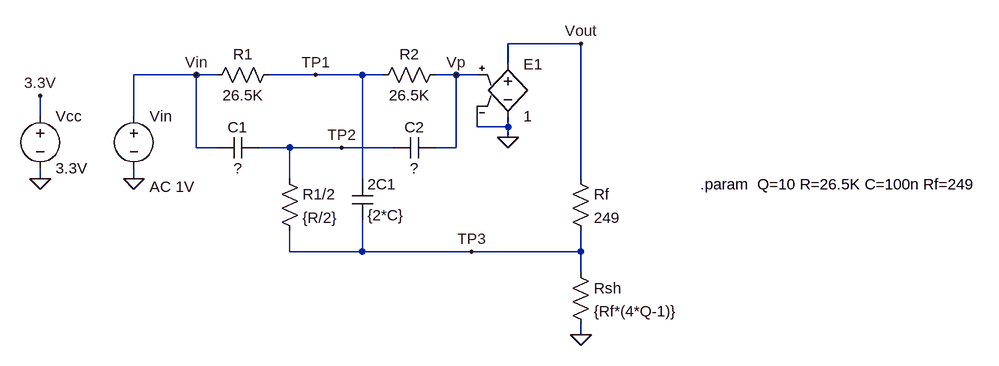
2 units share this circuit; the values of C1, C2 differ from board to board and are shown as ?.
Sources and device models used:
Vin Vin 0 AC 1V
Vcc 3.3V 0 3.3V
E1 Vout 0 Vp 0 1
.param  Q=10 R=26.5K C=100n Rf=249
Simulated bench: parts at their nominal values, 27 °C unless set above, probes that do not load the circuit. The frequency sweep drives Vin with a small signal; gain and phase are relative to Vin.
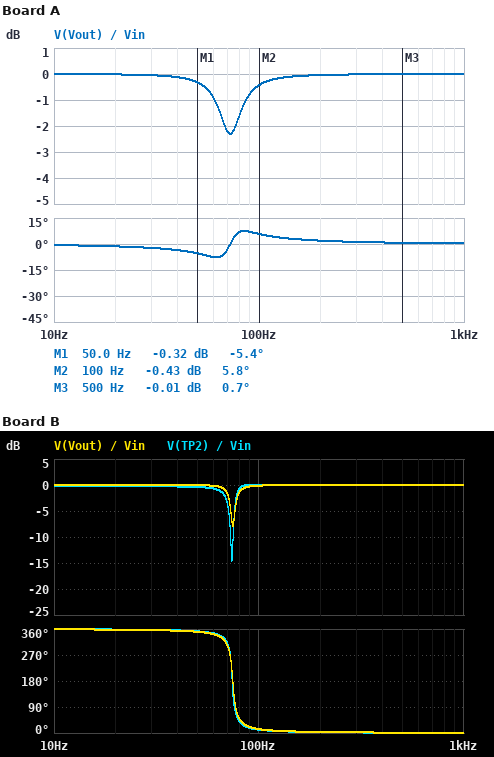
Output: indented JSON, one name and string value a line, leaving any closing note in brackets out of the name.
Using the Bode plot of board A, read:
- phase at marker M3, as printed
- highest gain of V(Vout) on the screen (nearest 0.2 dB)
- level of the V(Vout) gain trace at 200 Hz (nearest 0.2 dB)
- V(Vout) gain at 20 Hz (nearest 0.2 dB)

{
  "phase at marker M3, as printed": "0.7 deg",
  "highest gain of V(Vout) on the screen": "0 dB",
  "level of the V(Vout) gain trace at 200 Hz": "0 dB",
  "V(Vout) gain at 20 Hz": "0 dB"
}
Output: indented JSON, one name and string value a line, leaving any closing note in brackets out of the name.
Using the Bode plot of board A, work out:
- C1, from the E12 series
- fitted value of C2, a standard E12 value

{
  "C1, from the E12 series": "270 nF",
  "fitted value of C2, a standard E12 value": "33 nF"
}
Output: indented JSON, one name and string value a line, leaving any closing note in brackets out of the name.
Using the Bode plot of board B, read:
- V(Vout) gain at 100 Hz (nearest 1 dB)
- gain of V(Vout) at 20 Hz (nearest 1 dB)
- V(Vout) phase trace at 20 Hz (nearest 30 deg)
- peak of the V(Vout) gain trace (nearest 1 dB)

{
  "V(Vout) gain at 100 Hz": "0 dB",
  "gain of V(Vout) at 20 Hz": "0 dB",
  "V(Vout) phase trace at 20 Hz": "360 deg",
  "peak of the V(Vout) gain trace": "0 dB"
}
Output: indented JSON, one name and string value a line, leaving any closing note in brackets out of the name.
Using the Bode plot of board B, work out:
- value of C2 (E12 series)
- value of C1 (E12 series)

{
  "value of C2": "120 nF",
  "value of C1": "47 nF"
}
